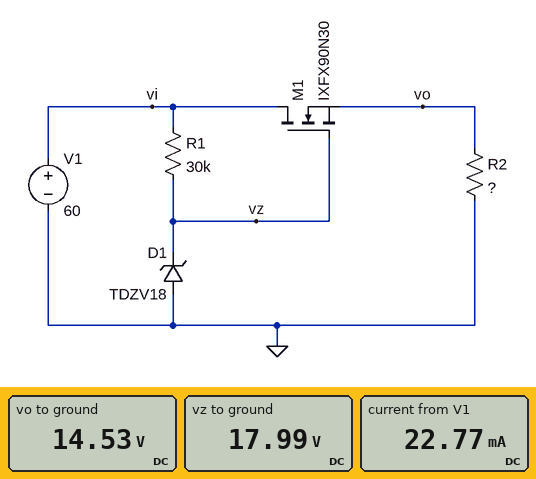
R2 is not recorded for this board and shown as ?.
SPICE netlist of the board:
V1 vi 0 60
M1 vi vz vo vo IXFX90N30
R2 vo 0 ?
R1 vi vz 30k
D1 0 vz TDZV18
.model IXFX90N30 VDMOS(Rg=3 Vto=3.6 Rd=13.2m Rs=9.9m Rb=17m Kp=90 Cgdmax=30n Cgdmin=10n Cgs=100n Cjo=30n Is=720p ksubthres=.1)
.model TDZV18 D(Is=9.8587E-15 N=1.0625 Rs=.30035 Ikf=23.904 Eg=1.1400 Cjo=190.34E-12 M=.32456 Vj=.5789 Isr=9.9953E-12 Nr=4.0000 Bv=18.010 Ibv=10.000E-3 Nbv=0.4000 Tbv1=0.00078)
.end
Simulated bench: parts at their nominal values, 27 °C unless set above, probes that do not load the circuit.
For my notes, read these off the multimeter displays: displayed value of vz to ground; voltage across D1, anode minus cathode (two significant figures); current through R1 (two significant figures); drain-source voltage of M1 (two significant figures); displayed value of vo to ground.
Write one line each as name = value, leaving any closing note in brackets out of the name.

displayed value of vz to ground = 17.99 V
voltage across D1, anode minus cathode = -18 V
current through R1 = 1.4 mA
drain-source voltage of M1 = 45 V
displayed value of vo to ground = 14.53 V
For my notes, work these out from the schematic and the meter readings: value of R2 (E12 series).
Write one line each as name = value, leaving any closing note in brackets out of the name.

value of R2 = 680 Ω
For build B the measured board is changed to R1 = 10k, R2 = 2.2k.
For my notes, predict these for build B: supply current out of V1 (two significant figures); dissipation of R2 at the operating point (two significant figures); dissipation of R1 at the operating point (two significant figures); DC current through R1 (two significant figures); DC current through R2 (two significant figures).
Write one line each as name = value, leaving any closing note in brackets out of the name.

supply current out of V1 = 11 mA
dissipation of R2 at the operating point = 97 mW
dissipation of R1 at the operating point = 180 mW
DC current through R1 = 4.2 mA
DC current through R2 = 6.6 mA
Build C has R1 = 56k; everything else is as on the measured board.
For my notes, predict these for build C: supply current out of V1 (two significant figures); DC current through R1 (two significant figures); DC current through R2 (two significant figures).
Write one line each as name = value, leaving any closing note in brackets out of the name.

supply current out of V1 = 22 mA
DC current through R1 = 750 µA
DC current through R2 = 21 mA
